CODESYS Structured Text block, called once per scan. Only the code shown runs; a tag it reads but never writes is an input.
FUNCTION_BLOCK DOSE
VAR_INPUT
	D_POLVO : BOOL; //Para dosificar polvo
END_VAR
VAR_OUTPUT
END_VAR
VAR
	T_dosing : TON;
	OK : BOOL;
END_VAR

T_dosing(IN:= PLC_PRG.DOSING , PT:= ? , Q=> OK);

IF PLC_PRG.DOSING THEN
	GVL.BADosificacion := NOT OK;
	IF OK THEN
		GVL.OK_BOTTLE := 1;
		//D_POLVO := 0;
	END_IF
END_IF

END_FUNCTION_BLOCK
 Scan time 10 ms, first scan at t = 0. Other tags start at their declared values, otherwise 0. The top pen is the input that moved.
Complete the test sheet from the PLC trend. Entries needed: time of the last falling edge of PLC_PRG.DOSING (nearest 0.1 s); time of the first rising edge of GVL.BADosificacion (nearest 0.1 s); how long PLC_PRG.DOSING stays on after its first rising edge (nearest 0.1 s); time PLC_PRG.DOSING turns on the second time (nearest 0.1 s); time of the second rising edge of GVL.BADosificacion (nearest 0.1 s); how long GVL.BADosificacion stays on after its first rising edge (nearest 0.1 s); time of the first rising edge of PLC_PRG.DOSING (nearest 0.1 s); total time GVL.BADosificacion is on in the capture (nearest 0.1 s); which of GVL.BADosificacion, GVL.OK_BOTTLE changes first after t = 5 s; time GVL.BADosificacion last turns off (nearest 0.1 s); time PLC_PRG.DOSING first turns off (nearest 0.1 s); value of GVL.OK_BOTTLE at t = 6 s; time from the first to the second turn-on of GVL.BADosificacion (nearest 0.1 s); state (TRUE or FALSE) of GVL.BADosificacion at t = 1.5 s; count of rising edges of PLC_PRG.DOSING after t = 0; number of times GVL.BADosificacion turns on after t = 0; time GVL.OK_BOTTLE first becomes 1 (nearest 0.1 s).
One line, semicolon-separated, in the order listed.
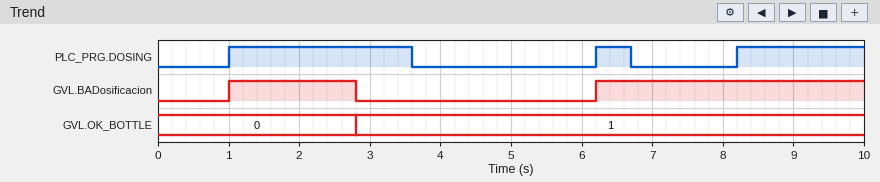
6.7 s; 1.0 s; 2.6 s; 6.2 s; 6.2 s; 1.8 s; 1.0 s; 5.6 s; GVL.BADosificacion; 2.8 s; 3.6 s; 1; 5.2 s; TRUE; 3; 2; 2.8 s
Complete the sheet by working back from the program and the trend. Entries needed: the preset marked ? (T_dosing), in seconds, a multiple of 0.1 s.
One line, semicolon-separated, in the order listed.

1.8 s
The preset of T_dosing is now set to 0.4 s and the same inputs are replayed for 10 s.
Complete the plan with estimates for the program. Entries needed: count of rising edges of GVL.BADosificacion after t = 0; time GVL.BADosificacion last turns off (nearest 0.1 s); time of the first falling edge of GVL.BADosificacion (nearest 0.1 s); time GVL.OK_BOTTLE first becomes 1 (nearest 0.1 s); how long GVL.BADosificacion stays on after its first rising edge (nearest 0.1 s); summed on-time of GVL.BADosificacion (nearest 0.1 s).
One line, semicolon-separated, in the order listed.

3; 8.6 s; 1.4 s; 1.4 s; 0.4 s; 1.2 s
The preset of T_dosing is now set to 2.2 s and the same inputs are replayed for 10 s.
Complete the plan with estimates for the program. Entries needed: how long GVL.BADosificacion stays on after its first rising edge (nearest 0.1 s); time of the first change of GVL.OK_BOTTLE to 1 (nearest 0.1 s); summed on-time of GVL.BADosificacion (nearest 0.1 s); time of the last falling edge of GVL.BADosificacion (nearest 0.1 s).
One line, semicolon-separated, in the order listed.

2.2 s; 3.2 s; 6.0 s; 3.2 s
